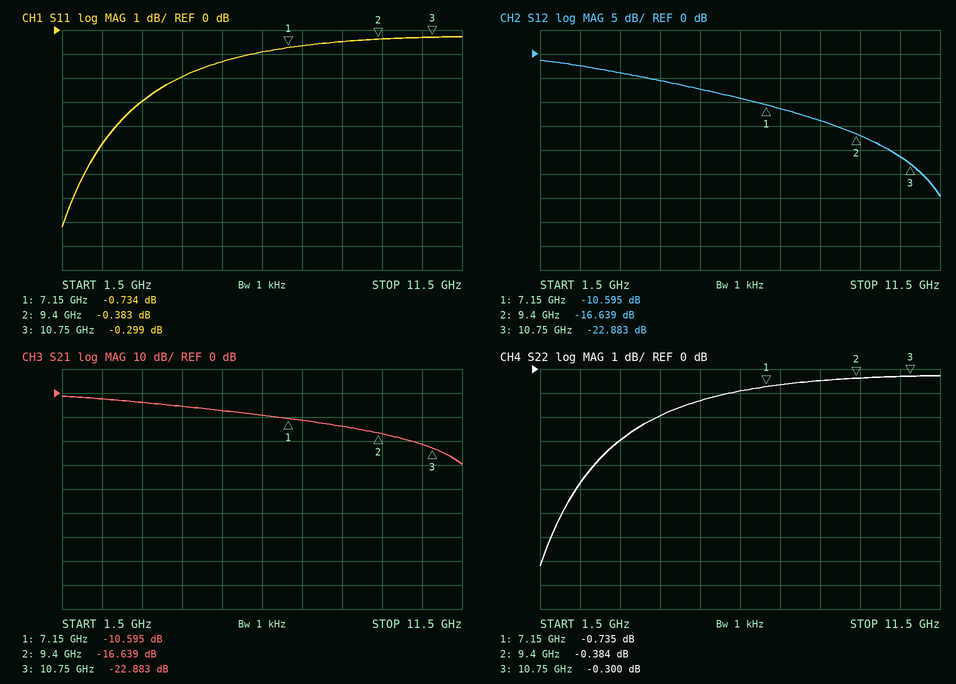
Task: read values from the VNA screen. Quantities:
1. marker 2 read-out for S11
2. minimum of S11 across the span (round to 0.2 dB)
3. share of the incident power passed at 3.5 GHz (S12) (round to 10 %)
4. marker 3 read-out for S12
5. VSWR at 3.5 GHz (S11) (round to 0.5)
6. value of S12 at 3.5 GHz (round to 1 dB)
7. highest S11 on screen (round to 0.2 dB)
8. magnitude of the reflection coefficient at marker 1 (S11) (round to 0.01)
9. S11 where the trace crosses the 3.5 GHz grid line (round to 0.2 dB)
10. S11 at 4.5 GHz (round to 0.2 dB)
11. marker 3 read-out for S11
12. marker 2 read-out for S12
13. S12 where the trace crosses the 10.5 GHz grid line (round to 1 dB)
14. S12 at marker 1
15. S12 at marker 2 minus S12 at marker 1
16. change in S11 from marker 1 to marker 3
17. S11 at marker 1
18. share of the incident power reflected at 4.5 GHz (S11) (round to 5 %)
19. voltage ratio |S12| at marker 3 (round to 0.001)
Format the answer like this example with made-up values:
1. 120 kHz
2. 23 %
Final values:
1. -0.383 dB
2. -8.2 dB
3. 40 %
4. -22.883 dB
5. 6.0
6. -4 dB
7. -0.2 dB
8. 0.92
9. -3.0 dB
10. -2.0 dB
11. -0.299 dB
12. -16.639 dB
13. -21 dB
14. -10.595 dB
15. -6.044 dB
16. 0.435 dB
17. -0.734 dB
18. 65 %
19. 0.072
